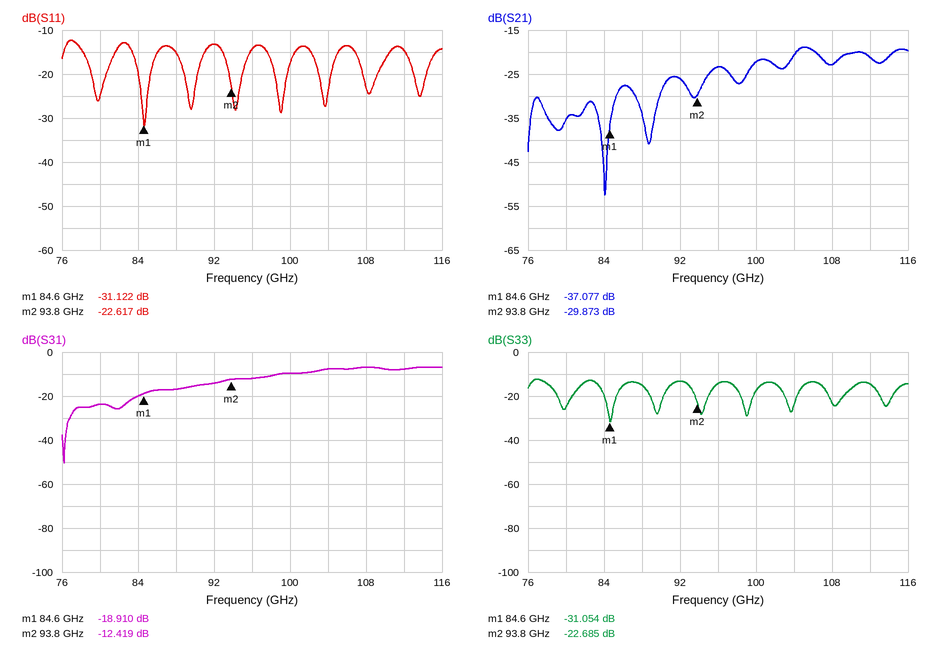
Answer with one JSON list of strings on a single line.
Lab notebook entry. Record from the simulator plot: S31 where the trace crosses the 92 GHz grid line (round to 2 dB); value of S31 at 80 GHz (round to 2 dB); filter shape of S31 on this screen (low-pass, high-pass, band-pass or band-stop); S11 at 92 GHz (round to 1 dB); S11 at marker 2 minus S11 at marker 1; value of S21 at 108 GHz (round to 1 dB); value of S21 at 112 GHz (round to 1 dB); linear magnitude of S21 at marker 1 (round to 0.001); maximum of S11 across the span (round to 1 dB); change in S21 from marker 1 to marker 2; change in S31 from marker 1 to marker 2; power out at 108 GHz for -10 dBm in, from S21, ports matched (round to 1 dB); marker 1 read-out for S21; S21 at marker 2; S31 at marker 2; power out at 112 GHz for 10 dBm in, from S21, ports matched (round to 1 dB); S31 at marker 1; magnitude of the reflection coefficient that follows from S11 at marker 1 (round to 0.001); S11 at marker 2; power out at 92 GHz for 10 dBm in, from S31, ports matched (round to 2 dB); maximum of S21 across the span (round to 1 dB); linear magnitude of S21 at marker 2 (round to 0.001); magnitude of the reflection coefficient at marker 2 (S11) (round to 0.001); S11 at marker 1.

["-14 dB", "-24 dB", "high-pass", "-13 dB", "8.505 dB", "-23 dB", "-21 dB", "0.014", "-12 dB", "7.204 dB", "6.491 dB", "-33 dBm", "-37.077 dB", "-29.873 dB", "-12.419 dB", "-11 dBm", "-18.910 dB", "0.028", "-22.617 dB", "-4 dBm", "-19 dB", "0.032", "0.074", "-31.122 dB"]
